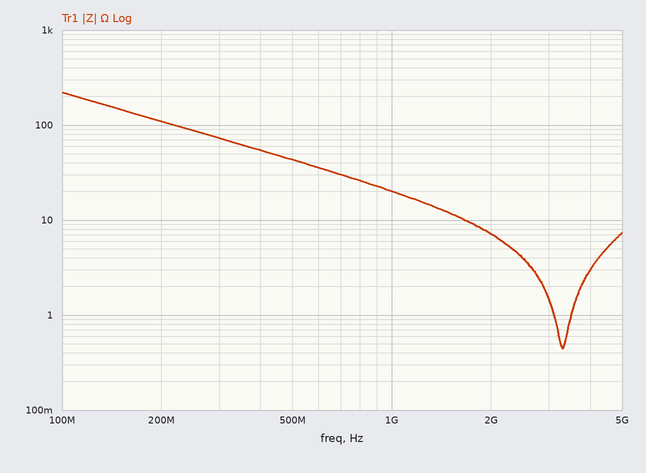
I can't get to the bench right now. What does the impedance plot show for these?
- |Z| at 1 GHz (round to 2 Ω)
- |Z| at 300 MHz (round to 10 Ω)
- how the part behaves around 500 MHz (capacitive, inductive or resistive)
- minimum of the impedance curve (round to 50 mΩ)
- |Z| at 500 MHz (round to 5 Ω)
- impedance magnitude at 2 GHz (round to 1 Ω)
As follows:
20 Ω
70 Ω
capacitive
450 mΩ
45 Ω
7 Ω
